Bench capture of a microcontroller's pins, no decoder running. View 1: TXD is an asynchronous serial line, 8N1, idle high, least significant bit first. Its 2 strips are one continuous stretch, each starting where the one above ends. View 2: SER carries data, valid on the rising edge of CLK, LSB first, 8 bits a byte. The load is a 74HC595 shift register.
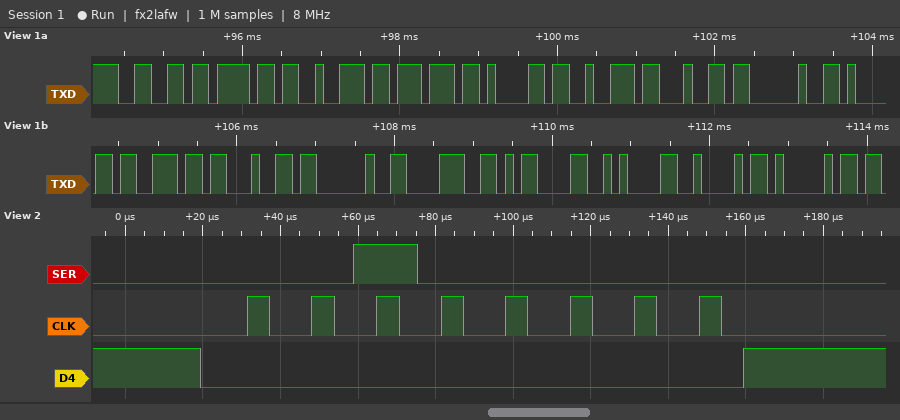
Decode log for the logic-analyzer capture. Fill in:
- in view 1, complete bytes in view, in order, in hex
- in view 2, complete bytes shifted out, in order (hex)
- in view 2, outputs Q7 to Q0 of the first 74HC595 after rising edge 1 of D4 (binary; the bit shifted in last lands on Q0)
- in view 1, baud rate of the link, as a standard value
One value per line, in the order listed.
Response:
0x66 0x6F 0x72 0x77 0x61 0x72 0x64 0x20 0x61 0x6E 0x64 0x20 0x38 0x0D 0x0A 0x42 0x41
04
00100000
9600 baud
